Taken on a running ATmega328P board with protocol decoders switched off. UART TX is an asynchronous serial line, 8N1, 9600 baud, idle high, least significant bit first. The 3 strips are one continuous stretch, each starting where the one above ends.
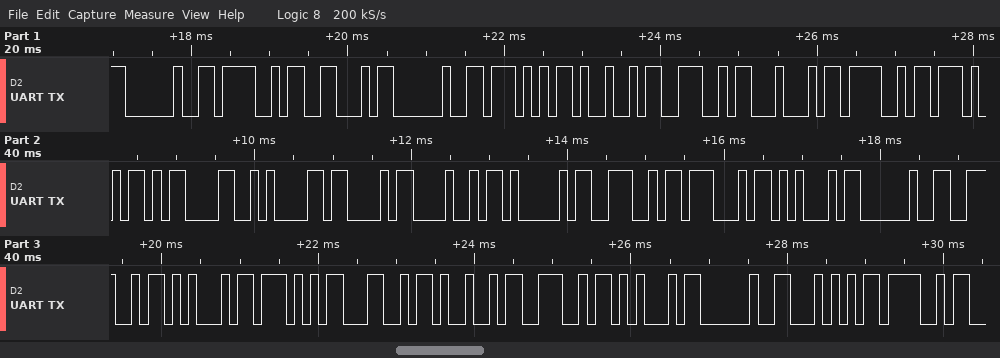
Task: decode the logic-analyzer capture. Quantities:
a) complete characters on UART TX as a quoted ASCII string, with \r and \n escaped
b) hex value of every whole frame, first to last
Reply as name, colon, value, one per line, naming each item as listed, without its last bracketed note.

complete characters on UART TX as a quoted ASCII string, with \r and \n escaped: " OF WINDOW\r\nCHANGE NEWLINE TO"
hex value of every whole frame, first to last: 20 4F 46 20 57 49 4E 44 4F 57 0D 0A 43 48 41 4E 47 45 20 4E 45 57 4C 49 4E 45 20 54 4F
